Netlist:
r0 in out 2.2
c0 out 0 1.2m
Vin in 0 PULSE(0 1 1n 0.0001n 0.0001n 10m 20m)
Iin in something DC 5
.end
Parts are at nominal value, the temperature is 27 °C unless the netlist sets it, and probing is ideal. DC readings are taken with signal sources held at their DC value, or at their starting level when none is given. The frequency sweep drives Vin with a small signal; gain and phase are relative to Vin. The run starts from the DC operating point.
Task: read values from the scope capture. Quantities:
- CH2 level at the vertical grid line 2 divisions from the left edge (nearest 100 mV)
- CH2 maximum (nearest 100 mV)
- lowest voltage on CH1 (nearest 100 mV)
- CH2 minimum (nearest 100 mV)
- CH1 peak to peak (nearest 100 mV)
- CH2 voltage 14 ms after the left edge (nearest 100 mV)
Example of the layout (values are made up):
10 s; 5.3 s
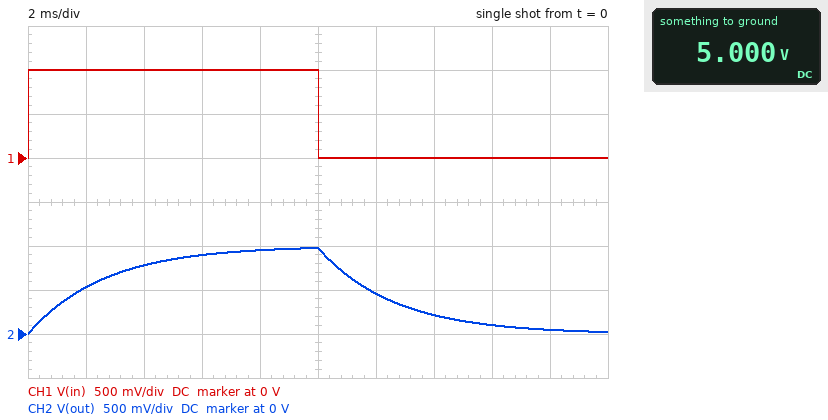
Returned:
800 mV; 1.0 V; 0 V; 0 V; 1.0 V; 200 mV
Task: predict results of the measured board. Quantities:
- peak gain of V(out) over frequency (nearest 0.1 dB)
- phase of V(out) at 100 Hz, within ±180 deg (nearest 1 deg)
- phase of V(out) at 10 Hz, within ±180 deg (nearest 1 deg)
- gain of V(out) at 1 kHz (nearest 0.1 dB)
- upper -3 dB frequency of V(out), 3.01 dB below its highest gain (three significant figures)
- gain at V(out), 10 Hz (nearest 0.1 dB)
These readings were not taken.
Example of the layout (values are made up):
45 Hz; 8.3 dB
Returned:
0 dB; -59 deg; -9 deg; -24.4 dB; 60.3 Hz; -0.1 dB
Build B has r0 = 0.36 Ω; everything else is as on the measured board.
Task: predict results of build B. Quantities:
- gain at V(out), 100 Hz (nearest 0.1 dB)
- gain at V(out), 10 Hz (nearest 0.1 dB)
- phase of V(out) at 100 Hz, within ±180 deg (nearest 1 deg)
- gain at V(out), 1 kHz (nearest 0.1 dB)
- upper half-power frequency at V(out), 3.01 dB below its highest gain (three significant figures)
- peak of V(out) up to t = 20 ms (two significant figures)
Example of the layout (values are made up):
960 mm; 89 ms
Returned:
-0.3 dB; 0 dB; -15 deg; -9.2 dB; 368 Hz; 1.0 V
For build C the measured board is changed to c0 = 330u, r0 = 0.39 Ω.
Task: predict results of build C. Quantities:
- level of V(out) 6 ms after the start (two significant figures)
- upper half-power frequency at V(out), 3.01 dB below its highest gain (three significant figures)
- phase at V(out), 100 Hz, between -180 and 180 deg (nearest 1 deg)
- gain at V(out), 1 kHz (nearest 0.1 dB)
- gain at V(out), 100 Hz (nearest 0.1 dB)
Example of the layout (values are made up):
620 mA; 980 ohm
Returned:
1.0 V; 1.24 kHz; -5 deg; -2.2 dB; 0 dB
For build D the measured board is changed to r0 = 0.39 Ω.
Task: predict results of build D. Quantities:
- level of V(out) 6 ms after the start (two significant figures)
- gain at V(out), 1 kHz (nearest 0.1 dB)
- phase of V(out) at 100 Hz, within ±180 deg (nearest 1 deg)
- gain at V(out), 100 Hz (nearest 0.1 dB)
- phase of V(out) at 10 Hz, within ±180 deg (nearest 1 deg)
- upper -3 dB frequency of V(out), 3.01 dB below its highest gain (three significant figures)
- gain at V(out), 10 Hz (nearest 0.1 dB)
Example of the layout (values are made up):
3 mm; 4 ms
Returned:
1.0 V; -9.8 dB; -16 deg; -0.4 dB; -2 deg; 340 Hz; 0 dB
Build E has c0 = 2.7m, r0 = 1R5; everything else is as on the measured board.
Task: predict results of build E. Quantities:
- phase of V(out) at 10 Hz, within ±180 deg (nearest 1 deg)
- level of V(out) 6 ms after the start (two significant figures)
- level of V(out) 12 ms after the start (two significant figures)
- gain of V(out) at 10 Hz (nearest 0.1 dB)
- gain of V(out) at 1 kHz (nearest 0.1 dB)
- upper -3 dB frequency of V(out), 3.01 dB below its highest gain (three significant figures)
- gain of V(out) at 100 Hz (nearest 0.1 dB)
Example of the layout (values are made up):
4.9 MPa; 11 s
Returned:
-14 deg; 770 mV; 560 mV; -0.3 dB; -28.1 dB; 39.3 Hz; -8.7 dB
